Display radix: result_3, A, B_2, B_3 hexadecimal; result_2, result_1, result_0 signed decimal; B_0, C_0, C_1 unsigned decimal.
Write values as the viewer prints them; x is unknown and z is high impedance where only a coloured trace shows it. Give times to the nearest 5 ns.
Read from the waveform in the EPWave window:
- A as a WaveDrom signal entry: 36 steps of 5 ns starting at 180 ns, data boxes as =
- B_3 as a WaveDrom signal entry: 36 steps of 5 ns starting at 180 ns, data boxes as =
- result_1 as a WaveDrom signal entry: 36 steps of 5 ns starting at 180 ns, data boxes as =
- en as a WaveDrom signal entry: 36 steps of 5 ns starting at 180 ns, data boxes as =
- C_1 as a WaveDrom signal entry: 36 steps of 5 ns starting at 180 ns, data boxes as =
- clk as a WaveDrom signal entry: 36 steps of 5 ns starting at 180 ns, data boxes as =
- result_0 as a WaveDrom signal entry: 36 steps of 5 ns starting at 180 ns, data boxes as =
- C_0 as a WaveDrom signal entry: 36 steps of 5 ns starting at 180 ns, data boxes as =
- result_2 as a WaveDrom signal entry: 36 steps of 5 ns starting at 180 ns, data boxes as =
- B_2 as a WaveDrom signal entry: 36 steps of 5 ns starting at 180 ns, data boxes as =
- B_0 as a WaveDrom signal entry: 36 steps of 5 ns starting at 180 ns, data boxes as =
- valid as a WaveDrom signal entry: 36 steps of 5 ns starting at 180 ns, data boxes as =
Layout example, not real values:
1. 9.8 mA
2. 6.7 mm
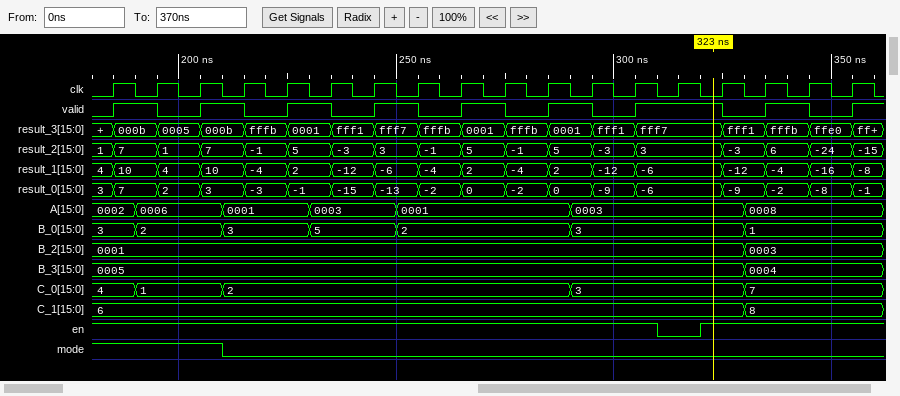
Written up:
1. {name: 'A', wave: '=.=...=...=...=.......=.......=.....', data: '0002 0006 0001 0003 0001 0003 0008'}
2. {name: 'B_3', wave: '=.............................=.....', data: '0005 0004'}
3. {name: 'result_1', wave: '==.=.=.=.=.=.=.=.=.=.=.=.=...=.=.=.=', data: '4 10 4 10 -4 2 -12 -6 -4 2 -4 2 -12 -6 -12 -4 -16 -8'}
4. {name: 'en', wave: '1.........................0.1.......'}
5. {name: 'C_1', wave: '=.............................=.....', data: '6 8'}
6. {name: 'clk', wave: '010101010101010101010101010101010101'}
7. {name: 'result_0', wave: '==.=.=.=.=.=.=.=.=.=.=.=.=...=.=.=.=', data: '3 7 2 3 -3 -1 -15 -13 -2 0 -2 0 -9 -6 -9 -2 -8 -1'}
8. {name: 'C_0', wave: '=.=...=...............=.......=.....', data: '4 1 2 3 7'}
9. {name: 'result_2', wave: '==.=.=.=.=.=.=.=.=.=.=.=.=...=.=.=.=', data: '1 7 1 7 -1 5 -3 3 -1 5 -1 5 -3 3 -3 6 -24 -15'}
10. {name: 'B_2', wave: '=.............................=.....', data: '0001 0003'}
11. {name: 'B_0', wave: '=.=...=...=...=.......=.......=.....', data: '3 2 3 5 2 3 1'}
12. {name: 'valid', wave: '01.0.1.0.1.0.1.0.1.0.1.0.1...0.1.0.1'}
